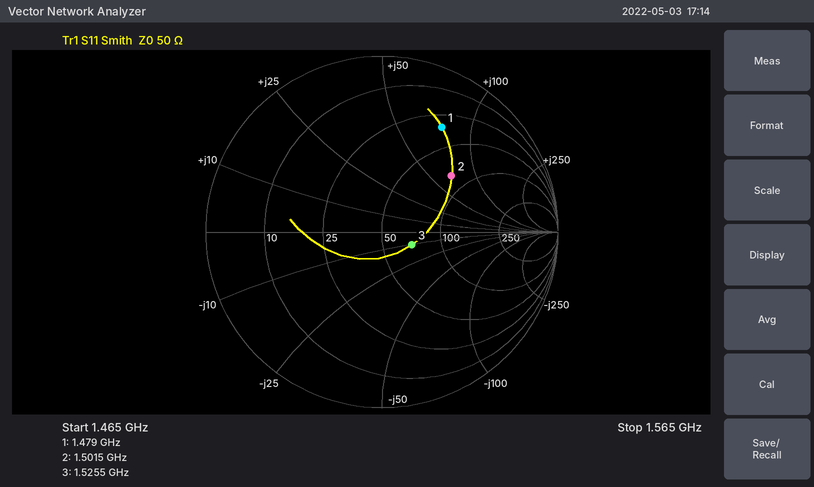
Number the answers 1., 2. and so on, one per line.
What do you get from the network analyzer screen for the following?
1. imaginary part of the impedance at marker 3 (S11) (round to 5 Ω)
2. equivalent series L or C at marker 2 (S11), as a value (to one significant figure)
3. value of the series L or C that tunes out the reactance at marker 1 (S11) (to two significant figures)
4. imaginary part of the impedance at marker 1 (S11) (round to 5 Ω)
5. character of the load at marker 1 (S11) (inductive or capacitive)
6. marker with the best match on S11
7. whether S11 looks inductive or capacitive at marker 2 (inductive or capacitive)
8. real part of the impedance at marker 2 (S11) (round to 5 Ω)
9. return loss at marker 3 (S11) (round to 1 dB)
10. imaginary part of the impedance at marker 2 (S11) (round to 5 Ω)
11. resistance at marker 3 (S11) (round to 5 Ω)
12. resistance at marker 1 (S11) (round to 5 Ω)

1. -10 Ω
2. 7 nH
3. 1.4 pF
4. +75 Ω
5. inductive
6. marker 3
7. inductive
8. 80 Ω
9. 15 dB
10. +70 Ω
11. 70 Ω
12. 35 Ω
